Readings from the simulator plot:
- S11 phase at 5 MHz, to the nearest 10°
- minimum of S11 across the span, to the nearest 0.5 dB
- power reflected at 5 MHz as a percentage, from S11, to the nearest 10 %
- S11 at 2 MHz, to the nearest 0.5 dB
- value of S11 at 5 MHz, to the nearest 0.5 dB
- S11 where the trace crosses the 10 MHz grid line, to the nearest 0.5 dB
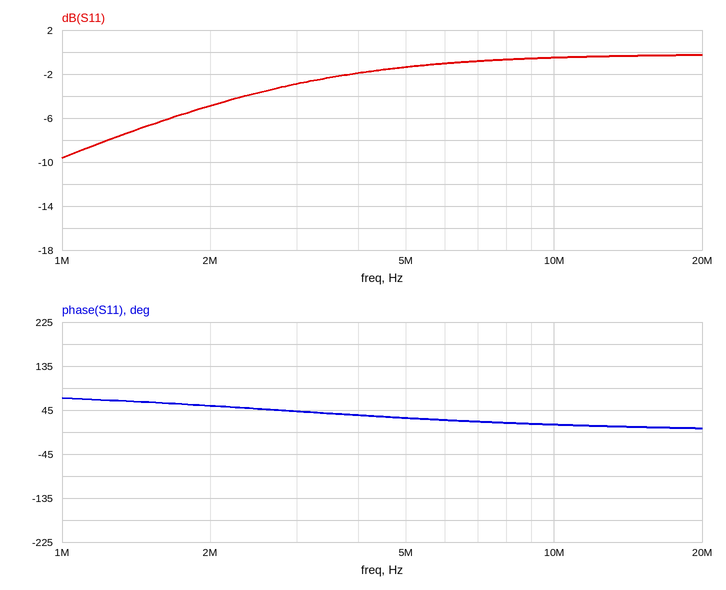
30°
-9.5 dB
70 %
-5.0 dB
-1.5 dB
-0.5 dB
